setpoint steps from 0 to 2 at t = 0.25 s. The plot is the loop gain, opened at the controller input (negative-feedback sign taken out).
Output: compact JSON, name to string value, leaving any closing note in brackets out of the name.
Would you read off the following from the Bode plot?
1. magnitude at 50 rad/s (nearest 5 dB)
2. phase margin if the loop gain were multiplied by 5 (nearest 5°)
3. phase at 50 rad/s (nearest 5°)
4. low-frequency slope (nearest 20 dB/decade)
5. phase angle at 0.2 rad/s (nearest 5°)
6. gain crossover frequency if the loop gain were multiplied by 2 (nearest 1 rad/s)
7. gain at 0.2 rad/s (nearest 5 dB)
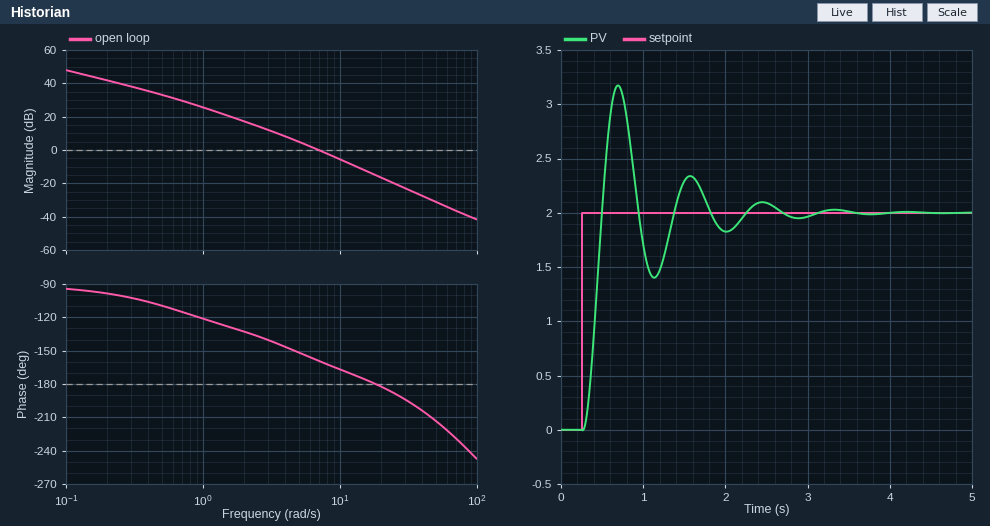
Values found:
{"magnitude at 50 rad/s": "-30 dB", "phase margin if the loop gain were multiplied by 5": "0°", "phase at 50 rad/s": "-215°", "low-frequency slope": "-20 dB/decade", "phase angle at 0.2 rad/s": "-100°", "gain crossover frequency if the loop gain were multiplied by 2": "10 rad/s", "gain at 0.2 rad/s": "40 dB"}
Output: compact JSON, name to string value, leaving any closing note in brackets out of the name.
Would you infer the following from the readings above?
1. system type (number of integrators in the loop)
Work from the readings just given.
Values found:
{"system type": "1"}
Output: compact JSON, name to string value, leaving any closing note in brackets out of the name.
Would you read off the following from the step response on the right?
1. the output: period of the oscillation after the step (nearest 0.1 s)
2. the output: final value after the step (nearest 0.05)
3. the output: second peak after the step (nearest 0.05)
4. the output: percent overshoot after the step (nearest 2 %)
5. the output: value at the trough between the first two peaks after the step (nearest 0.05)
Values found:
{"the output: period of the oscillation after the step": "0.9 s", "the output: final value after the step": "2.00", "the output: second peak after the step": "2.35", "the output: percent overshoot after the step": "58 %", "the output: value at the trough between the first two peaks after the step": "1.40"}
